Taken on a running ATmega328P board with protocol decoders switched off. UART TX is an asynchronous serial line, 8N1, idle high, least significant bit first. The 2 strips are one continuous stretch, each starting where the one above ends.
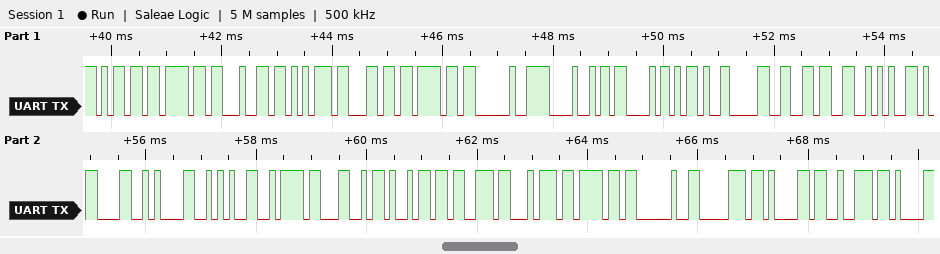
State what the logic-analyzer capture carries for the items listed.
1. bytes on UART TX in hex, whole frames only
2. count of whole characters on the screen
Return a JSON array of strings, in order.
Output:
["6D 6F 64 75 6C 6F 20 48 43 2D 30 36 2A 0D 0A 2A 7A 4C 69 73 74 6F 20 70 61 72", "26"]
